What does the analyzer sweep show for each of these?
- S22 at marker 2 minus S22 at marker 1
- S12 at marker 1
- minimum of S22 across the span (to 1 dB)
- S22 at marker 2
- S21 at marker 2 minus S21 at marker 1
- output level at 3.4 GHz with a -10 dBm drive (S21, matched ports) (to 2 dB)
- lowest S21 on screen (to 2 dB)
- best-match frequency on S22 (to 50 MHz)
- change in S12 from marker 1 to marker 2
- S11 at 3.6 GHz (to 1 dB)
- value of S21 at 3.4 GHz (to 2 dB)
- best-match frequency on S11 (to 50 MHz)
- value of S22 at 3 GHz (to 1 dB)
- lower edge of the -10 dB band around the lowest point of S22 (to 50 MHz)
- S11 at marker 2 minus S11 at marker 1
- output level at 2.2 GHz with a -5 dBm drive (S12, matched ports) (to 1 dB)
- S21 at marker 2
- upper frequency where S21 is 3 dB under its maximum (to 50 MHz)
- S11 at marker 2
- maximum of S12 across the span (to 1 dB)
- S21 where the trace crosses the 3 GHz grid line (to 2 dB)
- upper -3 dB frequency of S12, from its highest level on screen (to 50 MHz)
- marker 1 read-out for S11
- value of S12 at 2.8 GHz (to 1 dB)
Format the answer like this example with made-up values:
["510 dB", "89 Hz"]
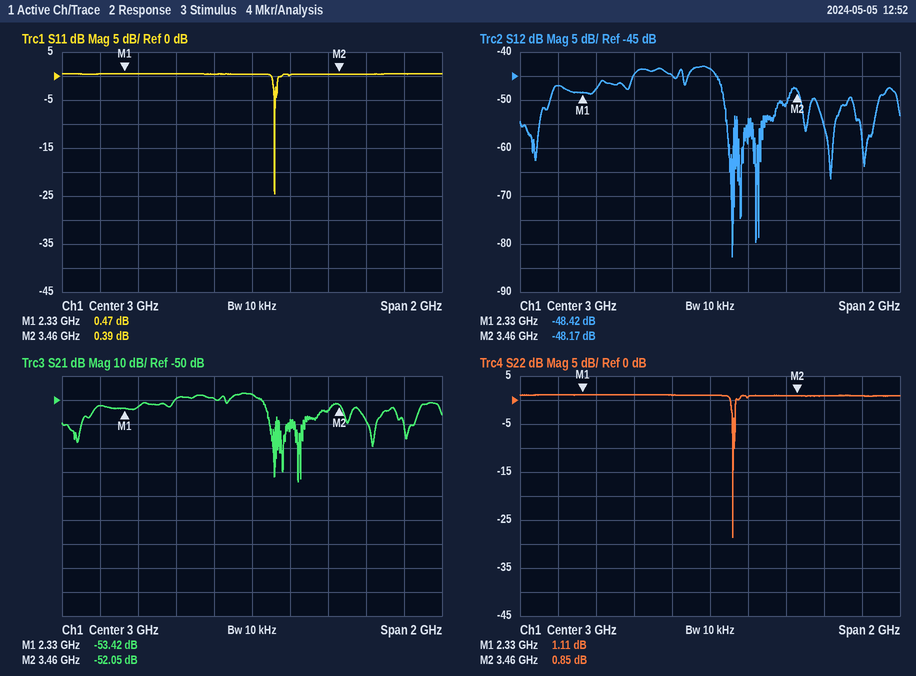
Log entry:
["-0.26 dB", "-48.42 dB", "-29 dB", "0.85 dB", "1.37 dB", "-64 dBm", "-84 dB", "3.10 GHz", "0.25 dB", "0 dB", "-54 dB", "3.10 GHz", "1 dB", "3.10 GHz", "-0.08 dB", "-52 dBm", "-52.05 dB", "3.05 GHz", "0.39 dB", "-43 dB", "-48 dB", "3.05 GHz", "0.47 dB", "-45 dB"]
